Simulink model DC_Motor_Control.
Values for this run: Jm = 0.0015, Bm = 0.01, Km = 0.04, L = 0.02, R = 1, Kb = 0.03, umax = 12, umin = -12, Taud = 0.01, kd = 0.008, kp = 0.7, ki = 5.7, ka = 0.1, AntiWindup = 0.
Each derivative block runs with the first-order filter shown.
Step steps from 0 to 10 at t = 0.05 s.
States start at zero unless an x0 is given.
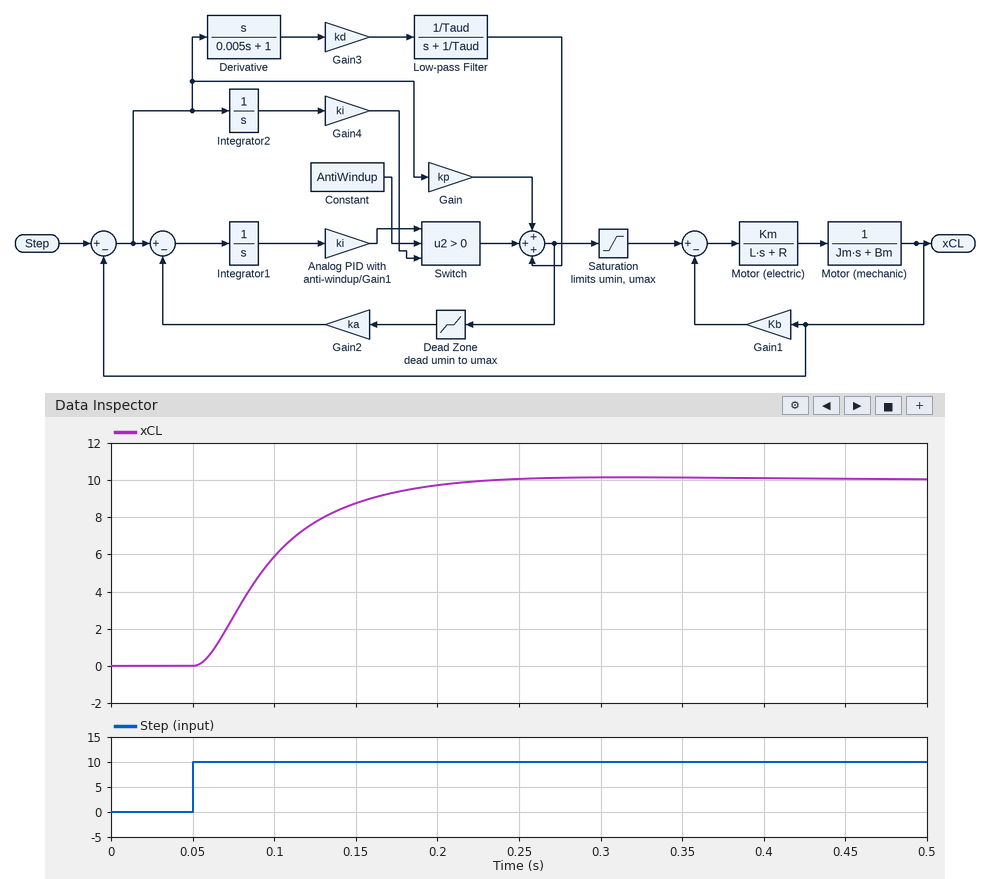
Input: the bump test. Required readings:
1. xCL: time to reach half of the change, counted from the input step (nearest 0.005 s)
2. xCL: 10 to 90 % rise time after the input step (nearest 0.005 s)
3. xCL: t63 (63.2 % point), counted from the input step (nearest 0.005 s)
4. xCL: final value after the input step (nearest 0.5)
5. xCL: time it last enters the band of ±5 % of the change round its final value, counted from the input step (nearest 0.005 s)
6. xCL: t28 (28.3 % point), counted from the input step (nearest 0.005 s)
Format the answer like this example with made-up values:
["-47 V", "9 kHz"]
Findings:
["0.040 s", "0.095 s", "0.055 s", "10.0", "0.135 s", "0.025 s"]
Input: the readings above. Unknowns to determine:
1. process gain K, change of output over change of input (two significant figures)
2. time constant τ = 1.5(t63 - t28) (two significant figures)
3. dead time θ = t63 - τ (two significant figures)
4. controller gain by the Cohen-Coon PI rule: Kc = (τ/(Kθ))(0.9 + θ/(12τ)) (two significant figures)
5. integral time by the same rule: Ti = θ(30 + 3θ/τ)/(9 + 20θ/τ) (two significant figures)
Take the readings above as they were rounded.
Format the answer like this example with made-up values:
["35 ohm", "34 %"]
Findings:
["1.0", "0.045 s", "0.010 s", "4.1", "0.023 s"]
